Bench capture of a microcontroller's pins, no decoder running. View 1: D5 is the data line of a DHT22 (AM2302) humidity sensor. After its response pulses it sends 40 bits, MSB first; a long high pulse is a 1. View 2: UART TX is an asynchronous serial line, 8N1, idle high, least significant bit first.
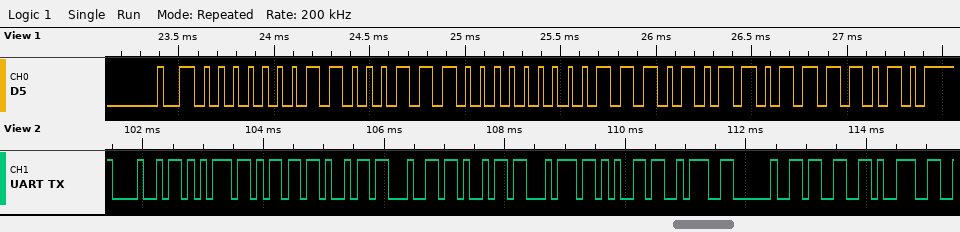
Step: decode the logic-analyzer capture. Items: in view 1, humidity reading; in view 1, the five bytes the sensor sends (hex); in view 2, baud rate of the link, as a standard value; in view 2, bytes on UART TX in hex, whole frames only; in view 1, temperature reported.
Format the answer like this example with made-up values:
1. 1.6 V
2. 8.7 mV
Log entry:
1. 39.8 %
2. 01 8E 00 EB 7A
3. 9600 baud
4. 0x48 0x75 0x6D 0x69 0x64 0x69 0x74 0x65 0x3A 0x20 0x33 0x39
5. 23.5 °C
